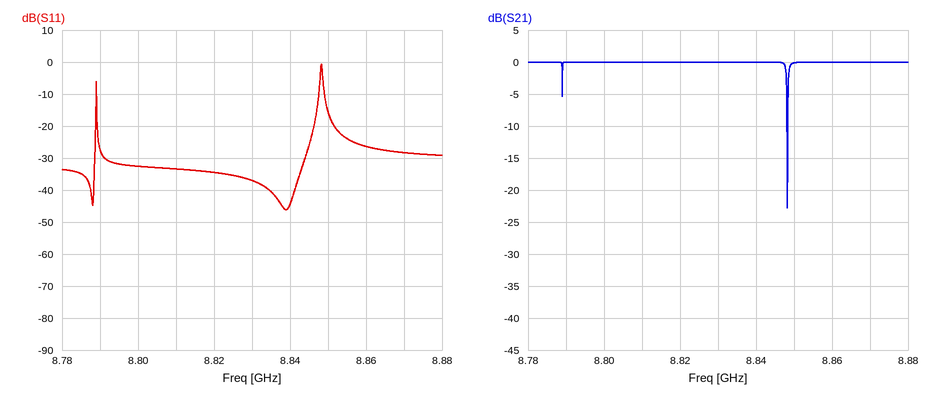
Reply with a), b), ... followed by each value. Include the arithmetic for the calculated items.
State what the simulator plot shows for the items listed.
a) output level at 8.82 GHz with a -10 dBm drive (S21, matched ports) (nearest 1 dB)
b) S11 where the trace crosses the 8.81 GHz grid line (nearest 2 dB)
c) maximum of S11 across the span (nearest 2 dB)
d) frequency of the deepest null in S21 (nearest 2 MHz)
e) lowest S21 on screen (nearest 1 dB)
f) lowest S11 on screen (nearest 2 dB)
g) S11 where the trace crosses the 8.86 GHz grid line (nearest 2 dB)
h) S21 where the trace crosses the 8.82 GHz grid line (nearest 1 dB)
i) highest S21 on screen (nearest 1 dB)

a) -10 dBm + (0 dB) = -10 dBm
b) -34 dB
c) 0 dB
d) 8.848 GHz
e) -23 dB
f) -46 dB
g) -26 dB
h) 0 dB
i) 0 dB
